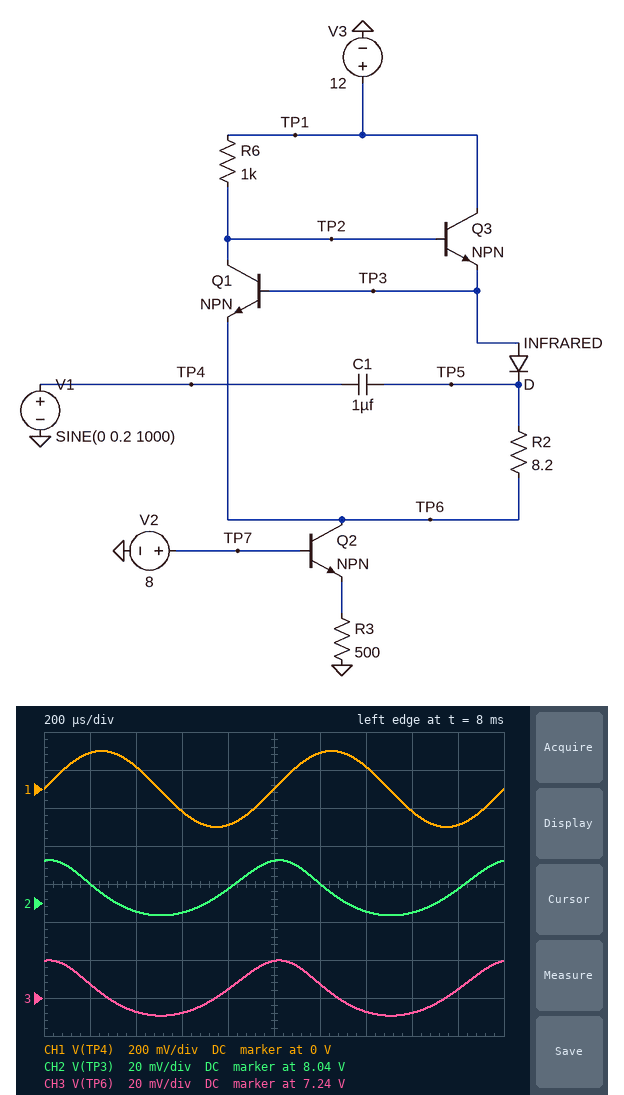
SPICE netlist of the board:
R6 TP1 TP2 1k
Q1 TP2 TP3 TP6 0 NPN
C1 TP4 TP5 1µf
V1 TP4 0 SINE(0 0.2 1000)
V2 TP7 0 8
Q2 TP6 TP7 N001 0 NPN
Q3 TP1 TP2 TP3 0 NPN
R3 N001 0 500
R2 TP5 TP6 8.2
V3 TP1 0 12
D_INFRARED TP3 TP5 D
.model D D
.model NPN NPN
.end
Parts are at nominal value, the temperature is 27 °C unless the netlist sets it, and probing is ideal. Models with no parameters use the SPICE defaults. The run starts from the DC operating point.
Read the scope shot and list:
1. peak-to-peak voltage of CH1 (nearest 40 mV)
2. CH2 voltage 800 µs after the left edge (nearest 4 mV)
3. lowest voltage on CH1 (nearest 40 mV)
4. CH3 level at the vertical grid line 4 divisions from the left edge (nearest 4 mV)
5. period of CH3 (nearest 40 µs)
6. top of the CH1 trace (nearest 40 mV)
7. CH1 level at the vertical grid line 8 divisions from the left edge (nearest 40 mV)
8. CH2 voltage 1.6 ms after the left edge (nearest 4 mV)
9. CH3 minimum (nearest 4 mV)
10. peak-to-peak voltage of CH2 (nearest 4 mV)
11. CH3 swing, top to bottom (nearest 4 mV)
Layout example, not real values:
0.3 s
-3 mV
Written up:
400 mV
8.048 V
-200 mV
7.244 V
1.00 ms
200 mV
-120 mV
8.036 V
7.232 V
28 mV
28 mV
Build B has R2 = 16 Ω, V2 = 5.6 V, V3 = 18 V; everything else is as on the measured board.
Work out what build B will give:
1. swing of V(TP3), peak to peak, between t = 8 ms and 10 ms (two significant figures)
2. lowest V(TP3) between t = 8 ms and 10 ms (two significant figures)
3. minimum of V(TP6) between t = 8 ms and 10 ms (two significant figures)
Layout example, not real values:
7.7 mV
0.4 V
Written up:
280 mV
14 V
13 V
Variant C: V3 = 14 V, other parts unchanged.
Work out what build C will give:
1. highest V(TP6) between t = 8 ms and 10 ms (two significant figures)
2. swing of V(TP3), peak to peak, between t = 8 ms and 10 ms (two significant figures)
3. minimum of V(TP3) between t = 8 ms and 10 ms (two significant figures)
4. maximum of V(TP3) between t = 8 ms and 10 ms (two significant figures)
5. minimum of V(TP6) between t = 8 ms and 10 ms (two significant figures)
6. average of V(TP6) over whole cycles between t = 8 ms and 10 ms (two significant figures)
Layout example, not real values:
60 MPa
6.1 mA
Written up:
9.1 V
260 mV
9.6 V
9.9 V
8.8 V
8.9 V
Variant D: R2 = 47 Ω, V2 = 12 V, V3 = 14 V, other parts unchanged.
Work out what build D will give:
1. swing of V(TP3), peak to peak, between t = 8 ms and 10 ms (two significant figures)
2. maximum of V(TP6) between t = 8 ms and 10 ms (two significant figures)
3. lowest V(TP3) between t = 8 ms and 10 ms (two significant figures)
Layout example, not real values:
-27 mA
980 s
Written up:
1.7 mV
11 V
12 V
